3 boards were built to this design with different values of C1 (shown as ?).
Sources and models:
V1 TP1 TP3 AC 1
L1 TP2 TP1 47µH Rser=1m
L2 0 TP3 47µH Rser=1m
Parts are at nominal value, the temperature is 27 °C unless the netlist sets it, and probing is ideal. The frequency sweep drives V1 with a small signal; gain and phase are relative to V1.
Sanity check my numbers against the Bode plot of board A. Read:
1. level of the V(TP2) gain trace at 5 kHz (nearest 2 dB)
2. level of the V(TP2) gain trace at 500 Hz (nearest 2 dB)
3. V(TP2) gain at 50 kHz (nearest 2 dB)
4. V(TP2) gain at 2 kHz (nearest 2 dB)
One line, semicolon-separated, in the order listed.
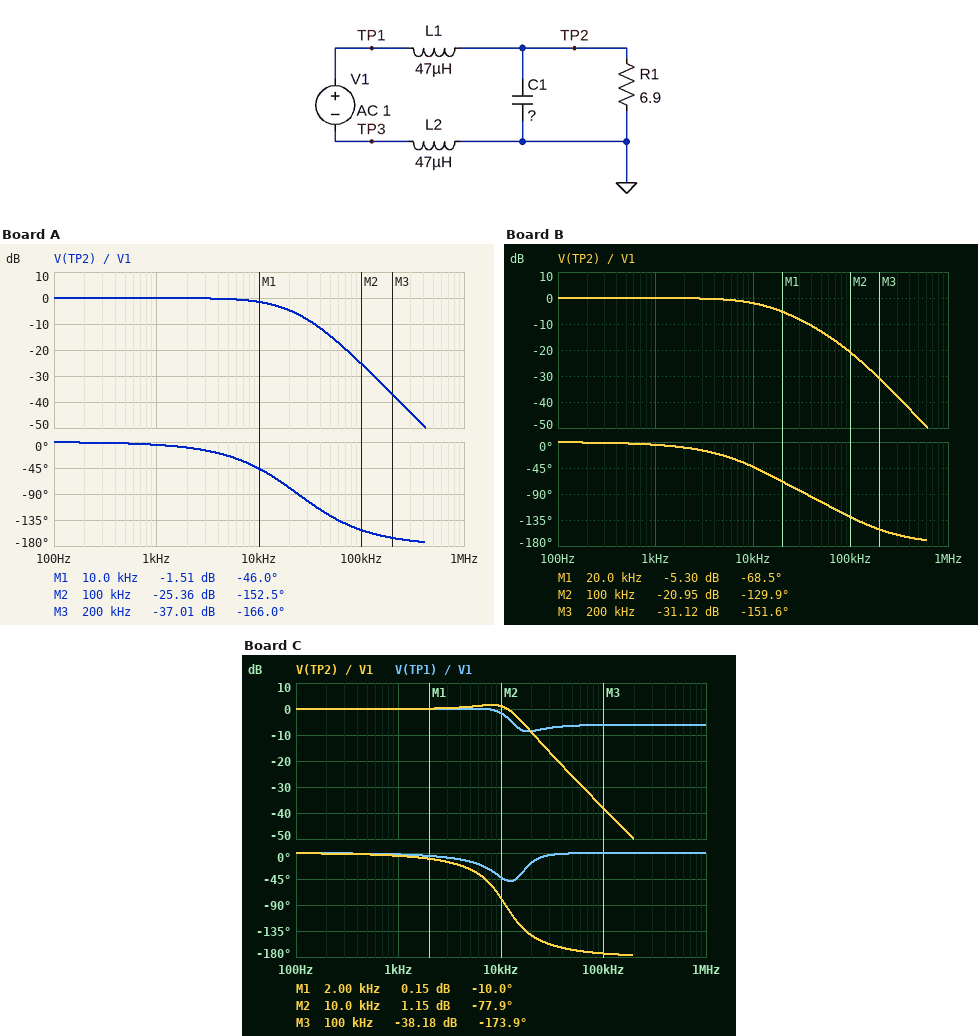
0 dB; 0 dB; -14 dB; 0 dB
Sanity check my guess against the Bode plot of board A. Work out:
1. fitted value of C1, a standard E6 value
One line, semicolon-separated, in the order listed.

470 nF
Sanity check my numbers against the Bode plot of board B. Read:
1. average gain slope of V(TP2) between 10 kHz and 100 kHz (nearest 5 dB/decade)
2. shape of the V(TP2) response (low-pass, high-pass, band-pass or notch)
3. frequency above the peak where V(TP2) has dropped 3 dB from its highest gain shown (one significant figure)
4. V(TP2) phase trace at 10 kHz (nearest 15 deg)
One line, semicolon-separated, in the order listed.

-20 dB/decade; low-pass; 10 kHz; -45 deg
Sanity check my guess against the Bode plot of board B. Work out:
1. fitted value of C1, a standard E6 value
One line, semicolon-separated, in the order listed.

220 nF
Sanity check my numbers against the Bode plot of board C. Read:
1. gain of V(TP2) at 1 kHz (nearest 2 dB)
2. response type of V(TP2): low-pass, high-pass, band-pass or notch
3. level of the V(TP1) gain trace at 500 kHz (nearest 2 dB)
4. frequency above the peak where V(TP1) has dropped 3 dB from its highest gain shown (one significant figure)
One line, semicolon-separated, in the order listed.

0 dB; low-pass; -6 dB; 10 kHz
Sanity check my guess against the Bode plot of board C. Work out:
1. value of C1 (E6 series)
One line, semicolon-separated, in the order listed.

2.2 µF
